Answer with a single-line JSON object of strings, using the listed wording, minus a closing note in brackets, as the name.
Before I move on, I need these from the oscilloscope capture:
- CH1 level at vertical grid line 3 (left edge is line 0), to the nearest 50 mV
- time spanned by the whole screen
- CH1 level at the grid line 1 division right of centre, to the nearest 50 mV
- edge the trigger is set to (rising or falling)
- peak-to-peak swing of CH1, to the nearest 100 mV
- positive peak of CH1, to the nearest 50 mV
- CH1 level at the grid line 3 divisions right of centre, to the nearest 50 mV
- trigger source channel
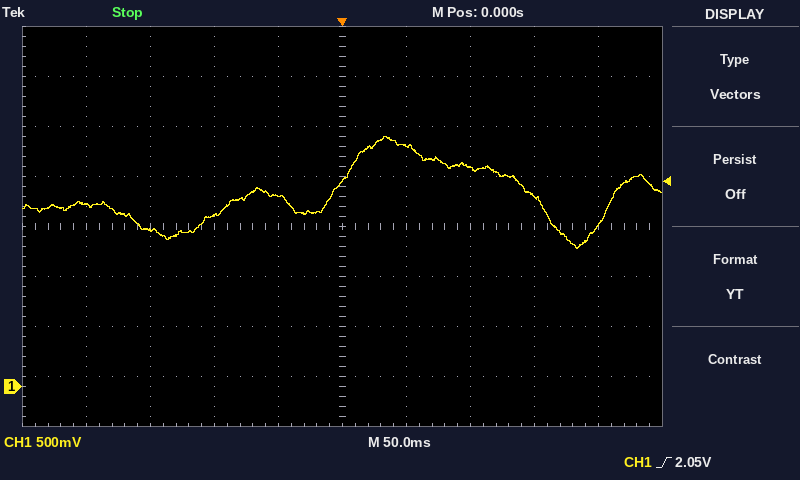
{"CH1 level at vertical grid line 3 (left edge is line 0), to the nearest 50 mV": "1.70 V", "time spanned by the whole screen": "500 ms", "CH1 level at the grid line 1 division right of centre, to the nearest 50 mV": "2.40 V", "edge the trigger is set to": "rising", "peak-to-peak swing of CH1, to the nearest 100 mV": "1.10 V", "positive peak of CH1, to the nearest 50 mV": "2.50 V", "CH1 level at the grid line 3 divisions right of centre, to the nearest 50 mV": "1.90 V", "trigger source channel": "CH1"}
